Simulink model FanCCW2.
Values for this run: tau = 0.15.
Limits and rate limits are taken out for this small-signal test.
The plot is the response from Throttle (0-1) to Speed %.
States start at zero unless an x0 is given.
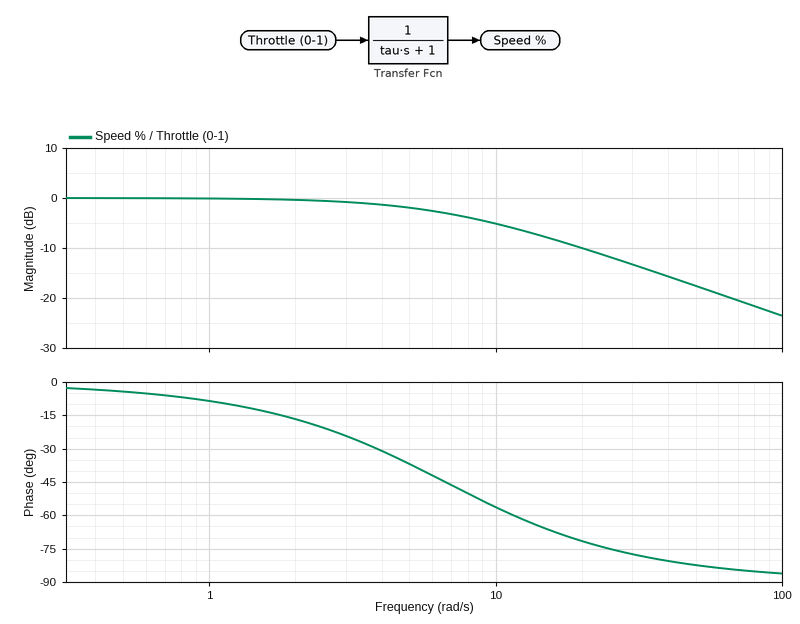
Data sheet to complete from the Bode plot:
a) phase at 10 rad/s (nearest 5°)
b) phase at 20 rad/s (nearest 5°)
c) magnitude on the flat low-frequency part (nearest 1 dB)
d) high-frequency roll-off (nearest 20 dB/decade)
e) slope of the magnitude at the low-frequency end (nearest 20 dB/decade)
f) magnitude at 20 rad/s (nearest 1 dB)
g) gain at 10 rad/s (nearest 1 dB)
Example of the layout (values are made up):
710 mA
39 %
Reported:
-55°
-70°
0 dB
-20 dB/decade
0 dB/decade
-10 dB
-5 dB
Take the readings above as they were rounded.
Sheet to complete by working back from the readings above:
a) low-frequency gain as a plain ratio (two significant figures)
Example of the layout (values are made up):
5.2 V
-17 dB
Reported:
1.0
